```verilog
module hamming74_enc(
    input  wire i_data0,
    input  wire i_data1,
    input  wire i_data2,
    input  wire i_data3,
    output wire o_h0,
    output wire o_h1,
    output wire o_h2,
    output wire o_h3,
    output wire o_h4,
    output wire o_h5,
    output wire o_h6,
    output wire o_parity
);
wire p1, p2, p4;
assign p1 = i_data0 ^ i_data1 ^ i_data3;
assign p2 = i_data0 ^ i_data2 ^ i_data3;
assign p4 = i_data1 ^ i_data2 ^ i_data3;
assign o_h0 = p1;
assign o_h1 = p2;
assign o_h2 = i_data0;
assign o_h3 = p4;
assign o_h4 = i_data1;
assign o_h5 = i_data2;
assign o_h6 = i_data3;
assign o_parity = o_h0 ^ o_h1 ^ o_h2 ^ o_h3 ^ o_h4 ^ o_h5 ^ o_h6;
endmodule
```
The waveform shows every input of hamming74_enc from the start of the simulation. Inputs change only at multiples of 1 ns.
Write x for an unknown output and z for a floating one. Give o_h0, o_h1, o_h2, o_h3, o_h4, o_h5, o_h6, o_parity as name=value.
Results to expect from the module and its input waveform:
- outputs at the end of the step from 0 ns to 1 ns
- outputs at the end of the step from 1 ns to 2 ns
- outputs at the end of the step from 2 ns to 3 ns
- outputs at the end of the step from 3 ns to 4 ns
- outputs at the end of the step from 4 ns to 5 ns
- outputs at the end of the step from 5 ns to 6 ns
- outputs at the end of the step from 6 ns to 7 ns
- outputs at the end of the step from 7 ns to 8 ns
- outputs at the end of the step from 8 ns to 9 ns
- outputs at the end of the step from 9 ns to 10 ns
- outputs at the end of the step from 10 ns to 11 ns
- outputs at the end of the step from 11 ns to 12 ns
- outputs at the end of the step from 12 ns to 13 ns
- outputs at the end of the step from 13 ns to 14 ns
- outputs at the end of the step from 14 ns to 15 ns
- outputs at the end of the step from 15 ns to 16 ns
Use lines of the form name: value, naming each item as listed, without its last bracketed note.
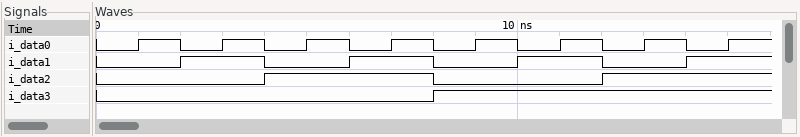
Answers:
outputs at the end of the step from 0 ns to 1 ns: o_h0=0, o_h1=0, o_h2=0, o_h3=0, o_h4=0, o_h5=0, o_h6=0, o_parity=0
outputs at the end of the step from 1 ns to 2 ns: o_h0=1, o_h1=1, o_h2=1, o_h3=0, o_h4=0, o_h5=0, o_h6=0, o_parity=1
outputs at the end of the step from 2 ns to 3 ns: o_h0=1, o_h1=0, o_h2=0, o_h3=1, o_h4=1, o_h5=0, o_h6=0, o_parity=1
outputs at the end of the step from 3 ns to 4 ns: o_h0=0, o_h1=1, o_h2=1, o_h3=1, o_h4=1, o_h5=0, o_h6=0, o_parity=0
outputs at the end of the step from 4 ns to 5 ns: o_h0=0, o_h1=1, o_h2=0, o_h3=1, o_h4=0, o_h5=1, o_h6=0, o_parity=1
outputs at the end of the step from 5 ns to 6 ns: o_h0=1, o_h1=0, o_h2=1, o_h3=1, o_h4=0, o_h5=1, o_h6=0, o_parity=0
outputs at the end of the step from 6 ns to 7 ns: o_h0=1, o_h1=1, o_h2=0, o_h3=0, o_h4=1, o_h5=1, o_h6=0, o_parity=0
outputs at the end of the step from 7 ns to 8 ns: o_h0=0, o_h1=0, o_h2=1, o_h3=0, o_h4=1, o_h5=1, o_h6=0, o_parity=1
outputs at the end of the step from 8 ns to 9 ns: o_h0=1, o_h1=1, o_h2=0, o_h3=1, o_h4=0, o_h5=0, o_h6=1, o_parity=0
outputs at the end of the step from 9 ns to 10 ns: o_h0=0, o_h1=0, o_h2=1, o_h3=1, o_h4=0, o_h5=0, o_h6=1, o_parity=1
outputs at the end of the step from 10 ns to 11 ns: o_h0=0, o_h1=1, o_h2=0, o_h3=0, o_h4=1, o_h5=0, o_h6=1, o_parity=1
outputs at the end of the step from 11 ns to 12 ns: o_h0=1, o_h1=0, o_h2=1, o_h3=0, o_h4=1, o_h5=0, o_h6=1, o_parity=0
outputs at the end of the step from 12 ns to 13 ns: o_h0=1, o_h1=0, o_h2=0, o_h3=0, o_h4=0, o_h5=1, o_h6=1, o_parity=1
outputs at the end of the step from 13 ns to 14 ns: o_h0=0, o_h1=1, o_h2=1, o_h3=0, o_h4=0, o_h5=1, o_h6=1, o_parity=0
outputs at the end of the step from 14 ns to 15 ns: o_h0=0, o_h1=0, o_h2=0, o_h3=1, o_h4=1, o_h5=1, o_h6=1, o_parity=0
outputs at the end of the step from 15 ns to 16 ns: o_h0=1, o_h1=1, o_h2=1, o_h3=1, o_h4=1, o_h5=1, o_h6=1, o_parity=1
